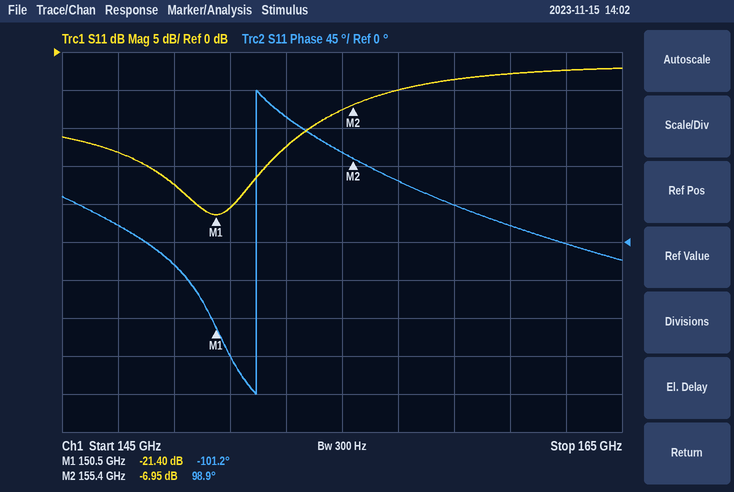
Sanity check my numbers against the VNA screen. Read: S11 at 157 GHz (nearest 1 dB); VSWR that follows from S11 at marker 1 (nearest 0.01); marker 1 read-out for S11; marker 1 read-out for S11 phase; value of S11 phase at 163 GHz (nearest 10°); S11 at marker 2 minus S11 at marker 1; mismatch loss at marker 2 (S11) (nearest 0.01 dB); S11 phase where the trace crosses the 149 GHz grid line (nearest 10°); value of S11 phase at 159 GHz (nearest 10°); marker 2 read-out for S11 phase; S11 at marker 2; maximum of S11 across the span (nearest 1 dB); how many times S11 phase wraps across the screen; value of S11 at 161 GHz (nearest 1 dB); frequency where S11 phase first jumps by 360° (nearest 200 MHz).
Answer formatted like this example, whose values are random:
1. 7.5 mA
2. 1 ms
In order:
1. -5 dB
2. 1.19
3. -21.40 dB
4. -101.2°
5. 0°
6. 14.45 dB
7. 0.98 dB
8. -30°
9. 40°
10. 98.9°
11. -6.95 dB
12. -2 dB
13. 1
14. -3 dB
15. 152.0 GHz
